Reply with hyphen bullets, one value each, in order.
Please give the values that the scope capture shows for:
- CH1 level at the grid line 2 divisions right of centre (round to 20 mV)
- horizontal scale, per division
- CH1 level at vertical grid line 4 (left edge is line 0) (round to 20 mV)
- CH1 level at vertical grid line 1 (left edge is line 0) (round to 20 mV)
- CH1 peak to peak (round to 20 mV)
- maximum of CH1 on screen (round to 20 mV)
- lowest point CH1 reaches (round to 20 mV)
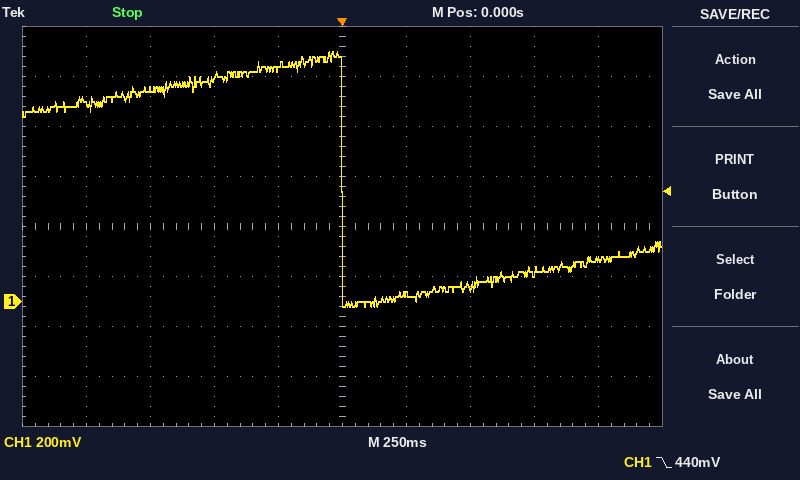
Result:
- 60 mV
- 250 ms
- 940 mV
- 800 mV
- 1.02 V
- 1.00 V
- -20 mV
